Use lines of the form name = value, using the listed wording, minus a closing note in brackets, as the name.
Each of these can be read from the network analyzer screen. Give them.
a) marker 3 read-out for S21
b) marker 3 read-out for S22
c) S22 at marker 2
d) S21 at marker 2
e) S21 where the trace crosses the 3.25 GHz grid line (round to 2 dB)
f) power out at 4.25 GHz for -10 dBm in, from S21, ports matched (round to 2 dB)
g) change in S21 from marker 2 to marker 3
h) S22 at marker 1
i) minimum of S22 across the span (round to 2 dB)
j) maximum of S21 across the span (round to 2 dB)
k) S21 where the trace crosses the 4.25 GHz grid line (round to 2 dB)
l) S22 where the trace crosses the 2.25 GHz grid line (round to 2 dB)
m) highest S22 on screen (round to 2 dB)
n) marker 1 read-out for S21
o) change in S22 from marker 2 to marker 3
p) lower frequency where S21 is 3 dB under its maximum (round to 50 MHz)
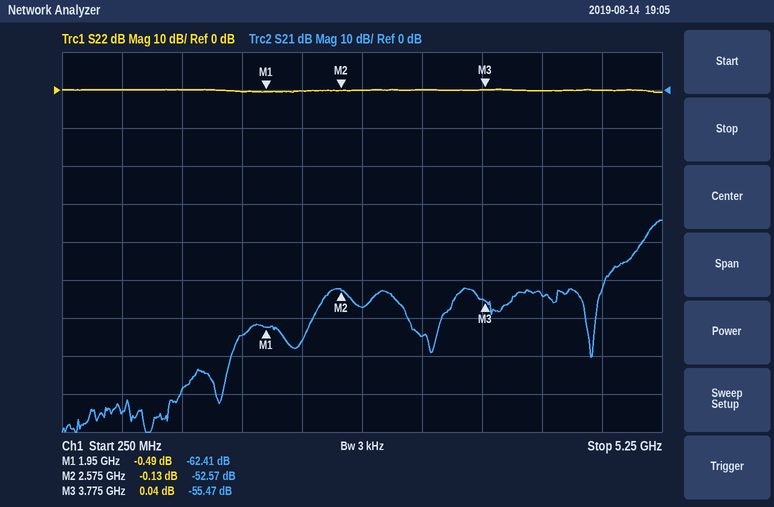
marker 3 read-out for S21 = -55.47 dB
marker 3 read-out for S22 = 0.04 dB
S22 at marker 2 = -0.13 dB
S21 at marker 2 = -52.57 dB
S21 where the trace crosses the 3.25 GHz grid line = -64 dB
power out at 4.25 GHz for -10 dBm in, from S21, ports matched = -64 dBm
change in S21 from marker 2 to marker 3 = -2.90 dB
S22 at marker 1 = -0.49 dB
minimum of S22 across the span = 0 dB
maximum of S21 across the span = -34 dB
S21 where the trace crosses the 4.25 GHz grid line = -54 dB
S22 where the trace crosses the 2.25 GHz grid line = 0 dB
highest S22 on screen = 0 dB
marker 1 read-out for S21 = -62.41 dB
change in S22 from marker 2 to marker 3 = 0.17 dB
lower frequency where S21 is 3 dB under its maximum = 5.15 GHz
